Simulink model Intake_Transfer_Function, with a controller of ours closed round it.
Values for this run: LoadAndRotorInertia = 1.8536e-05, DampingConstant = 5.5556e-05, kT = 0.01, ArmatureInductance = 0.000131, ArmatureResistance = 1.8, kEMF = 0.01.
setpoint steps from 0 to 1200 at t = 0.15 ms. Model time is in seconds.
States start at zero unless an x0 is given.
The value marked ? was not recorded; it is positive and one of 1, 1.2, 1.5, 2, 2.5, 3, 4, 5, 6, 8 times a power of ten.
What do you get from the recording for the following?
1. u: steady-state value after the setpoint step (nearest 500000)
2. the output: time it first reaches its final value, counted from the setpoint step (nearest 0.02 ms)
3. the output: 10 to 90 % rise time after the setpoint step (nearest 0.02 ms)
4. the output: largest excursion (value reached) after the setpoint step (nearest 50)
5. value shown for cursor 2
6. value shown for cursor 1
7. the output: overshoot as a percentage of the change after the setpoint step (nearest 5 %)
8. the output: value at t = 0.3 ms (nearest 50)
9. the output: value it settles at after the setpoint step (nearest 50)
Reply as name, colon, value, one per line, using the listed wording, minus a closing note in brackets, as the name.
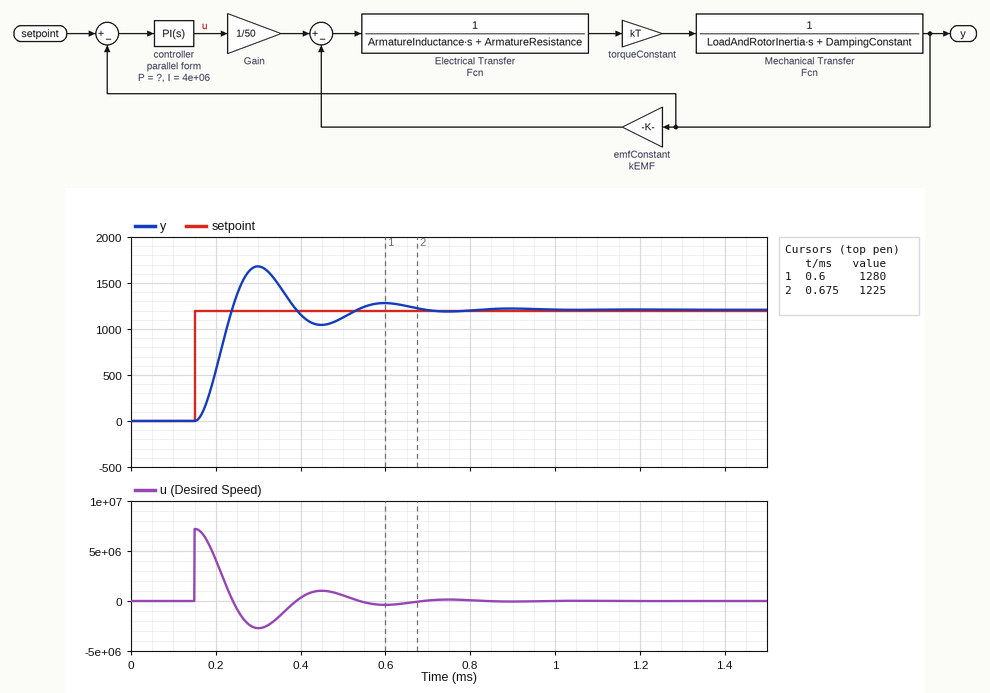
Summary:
u: steady-state value after the setpoint step: 0
the output: time it first reaches its final value, counted from the setpoint step: 0.08 ms
the output: 10 to 90 % rise time after the setpoint step: 0.06 ms
the output: largest excursion (value reached) after the setpoint step: 1700
value shown for cursor 2: 1225
value shown for cursor 1: 1280
the output: overshoot as a percentage of the change after the setpoint step: 40 %
the output: value at t = 0.3 ms: 1700
the output: value it settles at after the setpoint step: 1200
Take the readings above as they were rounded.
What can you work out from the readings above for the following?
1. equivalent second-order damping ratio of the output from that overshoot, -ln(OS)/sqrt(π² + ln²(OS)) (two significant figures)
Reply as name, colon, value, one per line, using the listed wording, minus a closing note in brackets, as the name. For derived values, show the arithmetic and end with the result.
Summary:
equivalent second-order damping ratio of the output from that overshoot, -ln(OS)/sqrt(π² + ln²(OS)): ln(0.4) = -0.916; 0.916 / sqrt(9.870 + 0.840) = 0.28
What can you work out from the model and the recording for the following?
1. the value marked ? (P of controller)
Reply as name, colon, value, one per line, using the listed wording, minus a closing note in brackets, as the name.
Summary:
the value marked ?: 6000
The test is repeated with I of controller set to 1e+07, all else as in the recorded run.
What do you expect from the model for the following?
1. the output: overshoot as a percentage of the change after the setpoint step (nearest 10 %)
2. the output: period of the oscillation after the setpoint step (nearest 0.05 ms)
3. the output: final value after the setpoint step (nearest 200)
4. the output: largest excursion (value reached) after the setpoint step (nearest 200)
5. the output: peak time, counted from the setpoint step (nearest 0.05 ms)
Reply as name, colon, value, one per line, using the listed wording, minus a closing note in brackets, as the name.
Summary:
the output: overshoot as a percentage of the change after the setpoint step: 50 %
the output: period of the oscillation after the setpoint step: 0.30 ms
the output: final value after the setpoint step: 1200
the output: largest excursion (value reached) after the setpoint step: 1800
the output: peak time, counted from the setpoint step: 0.15 ms
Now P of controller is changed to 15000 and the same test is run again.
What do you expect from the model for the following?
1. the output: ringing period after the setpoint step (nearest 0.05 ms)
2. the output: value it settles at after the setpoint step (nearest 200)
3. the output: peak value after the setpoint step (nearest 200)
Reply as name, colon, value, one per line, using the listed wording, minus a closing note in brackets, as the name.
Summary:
the output: ringing period after the setpoint step: 0.20 ms
the output: value it settles at after the setpoint step: 1200
the output: peak value after the setpoint step: 1800
